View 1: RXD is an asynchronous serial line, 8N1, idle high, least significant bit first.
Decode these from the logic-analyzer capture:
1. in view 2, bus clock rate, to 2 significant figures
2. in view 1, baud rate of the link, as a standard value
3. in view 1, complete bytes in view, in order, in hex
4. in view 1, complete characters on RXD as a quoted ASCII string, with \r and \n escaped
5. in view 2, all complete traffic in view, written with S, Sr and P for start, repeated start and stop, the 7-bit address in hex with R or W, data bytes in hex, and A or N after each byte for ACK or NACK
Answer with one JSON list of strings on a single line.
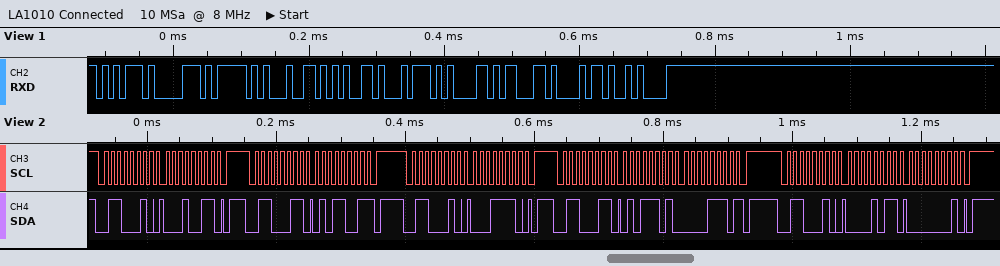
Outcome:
["100 kHz", "115200 baud", "0x75 0x70 0x5F 0x64 0x65 0x74 0x61 0x63 0x68 0x0A", "\"up_detach\\n\"", "S 31W A 13 A P S 31R A 59 N P S 31W A 1E A P S 31R A 5D A 0E N P S 31W A 0B A 01 A P"]
